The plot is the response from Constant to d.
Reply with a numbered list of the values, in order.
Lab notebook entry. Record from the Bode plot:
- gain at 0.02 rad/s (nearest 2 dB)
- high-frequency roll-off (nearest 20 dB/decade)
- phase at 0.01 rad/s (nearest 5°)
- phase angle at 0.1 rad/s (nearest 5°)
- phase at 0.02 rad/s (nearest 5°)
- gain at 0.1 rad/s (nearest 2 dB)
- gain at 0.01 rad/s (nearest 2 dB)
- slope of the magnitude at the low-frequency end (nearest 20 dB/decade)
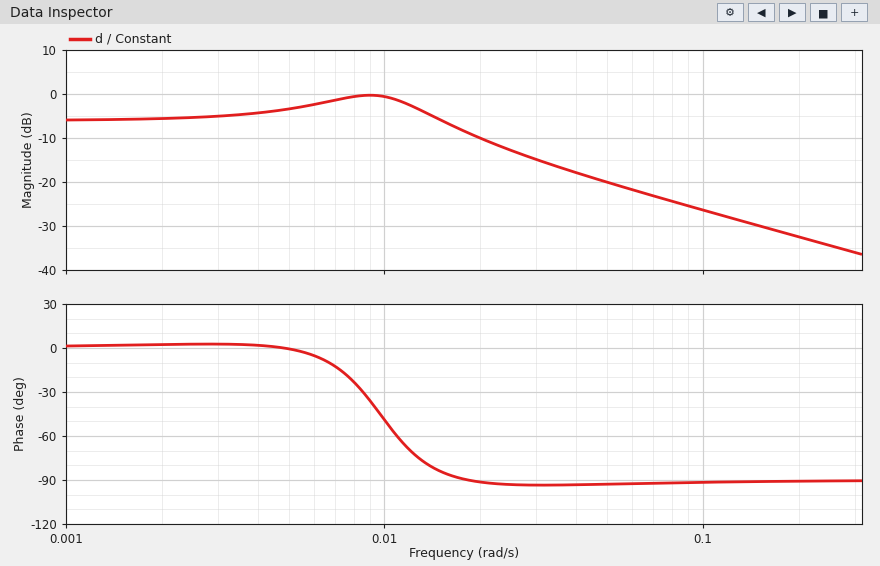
1. -10 dB
2. -20 dB/decade
3. -50°
4. -90°
5. -90°
6. -26 dB
7. 0 dB
8. 0 dB/decade
